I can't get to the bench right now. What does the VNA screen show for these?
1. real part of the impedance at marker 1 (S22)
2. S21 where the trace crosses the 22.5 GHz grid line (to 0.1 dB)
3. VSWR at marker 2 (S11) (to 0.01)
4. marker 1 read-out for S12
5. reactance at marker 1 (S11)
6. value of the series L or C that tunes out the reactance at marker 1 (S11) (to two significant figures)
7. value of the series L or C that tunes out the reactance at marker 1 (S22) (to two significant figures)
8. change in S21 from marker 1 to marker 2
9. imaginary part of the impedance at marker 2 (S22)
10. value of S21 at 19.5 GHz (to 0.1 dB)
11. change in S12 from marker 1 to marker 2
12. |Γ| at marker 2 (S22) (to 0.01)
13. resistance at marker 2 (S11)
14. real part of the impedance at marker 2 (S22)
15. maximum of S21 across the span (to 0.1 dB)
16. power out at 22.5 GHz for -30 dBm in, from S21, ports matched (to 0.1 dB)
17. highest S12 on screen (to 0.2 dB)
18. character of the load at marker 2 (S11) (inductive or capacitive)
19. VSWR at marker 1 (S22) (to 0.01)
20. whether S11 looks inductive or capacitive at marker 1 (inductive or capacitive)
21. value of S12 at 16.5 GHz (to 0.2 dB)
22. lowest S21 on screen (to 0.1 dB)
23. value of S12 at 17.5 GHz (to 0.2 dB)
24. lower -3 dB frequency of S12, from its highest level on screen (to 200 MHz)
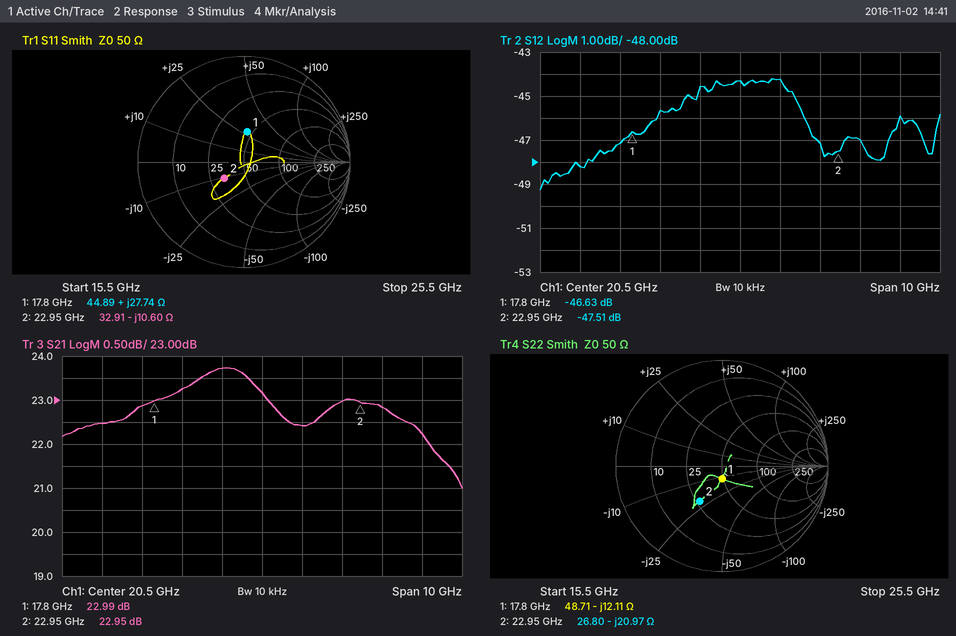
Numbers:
48.71 Ω
23.0 dB
1.63
-46.63 dB
+27.74 Ω
320 fF
110 pH
-0.04 dB
-20.97 Ω
23.7 dB
-0.88 dB
0.39
32.91 Ω
26.80 Ω
23.7 dB
-7.0 dBm
-44.2 dB
capacitive
1.28
inductive
-48.2 dB
21.0 dB
-47.2 dB
17.4 GHz
